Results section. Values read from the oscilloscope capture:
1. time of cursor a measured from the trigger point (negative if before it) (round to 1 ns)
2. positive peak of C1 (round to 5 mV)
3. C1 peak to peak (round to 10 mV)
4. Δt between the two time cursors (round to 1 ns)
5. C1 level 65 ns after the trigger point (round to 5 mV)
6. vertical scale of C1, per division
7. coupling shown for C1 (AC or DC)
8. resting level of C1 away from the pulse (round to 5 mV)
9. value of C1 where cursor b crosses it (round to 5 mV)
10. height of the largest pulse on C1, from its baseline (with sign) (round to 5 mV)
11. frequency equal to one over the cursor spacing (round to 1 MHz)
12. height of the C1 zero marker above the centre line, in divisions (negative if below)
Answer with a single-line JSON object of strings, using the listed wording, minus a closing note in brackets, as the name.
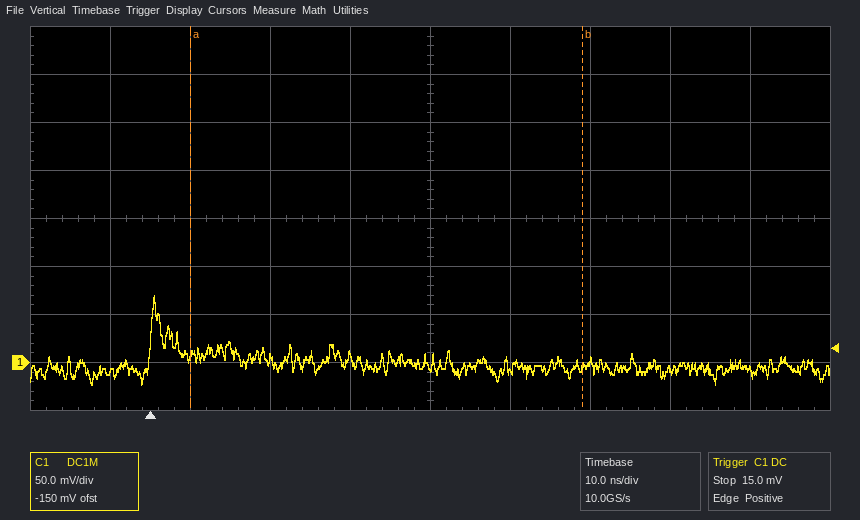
{"time of cursor a measured from the trigger point (negative if before it)": "+5 ns", "positive peak of C1": "70 mV", "C1 peak to peak": "90 mV", "Δt between the two time cursors": "49 ns", "C1 level 65 ns after the trigger point": "-10 mV", "vertical scale of C1, per division": "50 mV", "coupling shown for C1": "DC", "resting level of C1 away from the pulse": "-5 mV", "value of C1 where cursor b crosses it": "-5 mV", "height of the largest pulse on C1, from its baseline (with sign)": "+75 mV", "frequency equal to one over the cursor spacing": "20 MHz", "height of the C1 zero marker above the centre line, in divisions": "-3.0 div"}
